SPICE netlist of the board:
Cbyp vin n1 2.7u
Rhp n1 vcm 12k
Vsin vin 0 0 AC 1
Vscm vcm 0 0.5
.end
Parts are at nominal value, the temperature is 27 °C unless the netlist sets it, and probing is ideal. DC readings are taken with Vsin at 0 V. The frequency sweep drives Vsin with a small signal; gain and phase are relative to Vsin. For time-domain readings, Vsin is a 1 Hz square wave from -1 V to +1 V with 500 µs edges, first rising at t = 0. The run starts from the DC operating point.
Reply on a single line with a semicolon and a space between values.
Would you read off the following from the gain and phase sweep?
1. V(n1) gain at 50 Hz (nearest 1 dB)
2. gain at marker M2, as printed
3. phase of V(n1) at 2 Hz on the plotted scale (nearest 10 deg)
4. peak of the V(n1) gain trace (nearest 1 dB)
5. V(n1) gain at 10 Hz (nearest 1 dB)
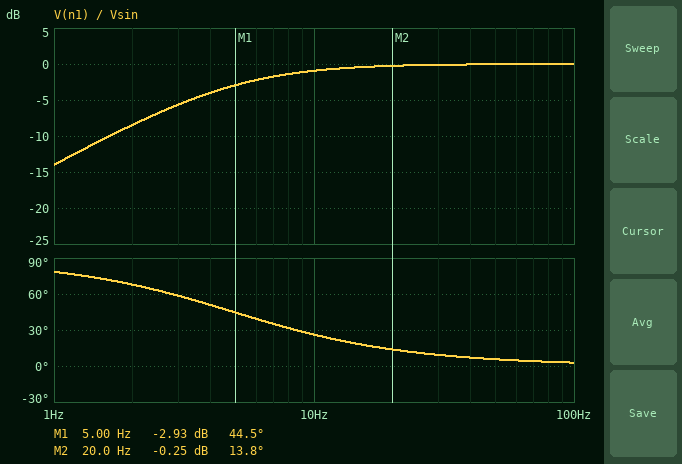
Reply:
0 dB; -0.25 dB; 70 deg; 0 dB; -1 dB
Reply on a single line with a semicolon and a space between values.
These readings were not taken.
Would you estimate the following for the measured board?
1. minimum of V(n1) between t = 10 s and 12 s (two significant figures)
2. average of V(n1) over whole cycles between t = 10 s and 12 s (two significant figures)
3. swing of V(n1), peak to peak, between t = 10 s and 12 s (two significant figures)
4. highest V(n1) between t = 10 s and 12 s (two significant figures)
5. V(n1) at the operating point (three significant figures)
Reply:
-1.5 V; 500 mV; 4.0 V; 2.5 V; 500 mV
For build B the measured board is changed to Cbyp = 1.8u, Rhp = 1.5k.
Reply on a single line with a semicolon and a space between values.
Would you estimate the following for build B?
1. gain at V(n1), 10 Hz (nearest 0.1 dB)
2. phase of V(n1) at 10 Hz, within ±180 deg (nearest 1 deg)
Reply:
-15.5 dB; 80 deg
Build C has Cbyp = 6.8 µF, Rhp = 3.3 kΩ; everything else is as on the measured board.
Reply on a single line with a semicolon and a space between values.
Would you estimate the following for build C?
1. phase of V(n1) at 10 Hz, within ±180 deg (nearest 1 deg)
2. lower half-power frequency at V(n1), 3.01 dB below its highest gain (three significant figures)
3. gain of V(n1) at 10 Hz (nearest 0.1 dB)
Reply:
35 deg; 7.09 Hz; -1.8 dB
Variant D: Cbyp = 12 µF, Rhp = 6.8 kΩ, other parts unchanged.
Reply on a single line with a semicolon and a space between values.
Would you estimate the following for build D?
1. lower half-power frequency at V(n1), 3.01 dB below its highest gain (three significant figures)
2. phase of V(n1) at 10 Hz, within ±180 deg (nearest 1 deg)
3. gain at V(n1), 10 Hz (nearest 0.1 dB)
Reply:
1.95 Hz; 11 deg; -0.2 dB
